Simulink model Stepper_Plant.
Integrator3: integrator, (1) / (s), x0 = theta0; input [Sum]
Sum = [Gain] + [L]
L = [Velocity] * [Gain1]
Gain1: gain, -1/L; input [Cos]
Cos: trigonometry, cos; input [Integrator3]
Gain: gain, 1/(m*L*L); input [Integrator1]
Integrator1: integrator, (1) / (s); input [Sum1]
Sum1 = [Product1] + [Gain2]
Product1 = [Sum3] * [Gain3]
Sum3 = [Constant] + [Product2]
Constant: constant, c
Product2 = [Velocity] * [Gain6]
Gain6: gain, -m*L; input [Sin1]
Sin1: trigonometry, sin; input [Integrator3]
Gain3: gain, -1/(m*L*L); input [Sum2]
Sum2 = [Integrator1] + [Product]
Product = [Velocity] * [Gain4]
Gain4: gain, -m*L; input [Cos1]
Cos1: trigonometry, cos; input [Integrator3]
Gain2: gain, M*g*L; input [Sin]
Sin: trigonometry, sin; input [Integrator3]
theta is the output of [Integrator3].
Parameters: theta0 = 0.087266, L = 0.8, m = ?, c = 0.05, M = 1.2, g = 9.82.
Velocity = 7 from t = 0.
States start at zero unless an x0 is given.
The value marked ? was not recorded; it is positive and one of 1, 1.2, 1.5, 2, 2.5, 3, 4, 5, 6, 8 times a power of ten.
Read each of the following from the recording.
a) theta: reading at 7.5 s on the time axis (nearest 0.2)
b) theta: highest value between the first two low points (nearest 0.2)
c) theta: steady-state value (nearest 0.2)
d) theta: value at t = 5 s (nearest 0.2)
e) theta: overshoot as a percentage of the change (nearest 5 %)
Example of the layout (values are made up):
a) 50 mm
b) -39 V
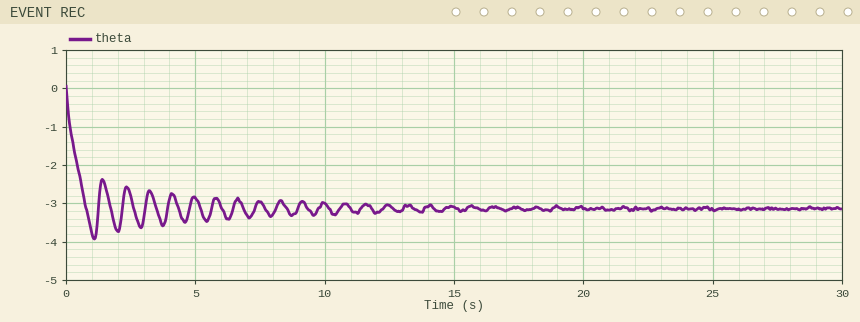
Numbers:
a) -3.0
b) -2.4
c) -3.2
d) -2.8
e) 25 %
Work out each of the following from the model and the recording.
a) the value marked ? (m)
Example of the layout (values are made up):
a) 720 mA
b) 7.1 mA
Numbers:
a) 0.25
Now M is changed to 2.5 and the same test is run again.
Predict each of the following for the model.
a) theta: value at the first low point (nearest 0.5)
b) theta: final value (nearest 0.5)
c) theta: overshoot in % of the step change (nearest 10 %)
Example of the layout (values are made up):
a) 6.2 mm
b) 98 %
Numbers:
a) -4.5
b) -3.0
c) 40 %
